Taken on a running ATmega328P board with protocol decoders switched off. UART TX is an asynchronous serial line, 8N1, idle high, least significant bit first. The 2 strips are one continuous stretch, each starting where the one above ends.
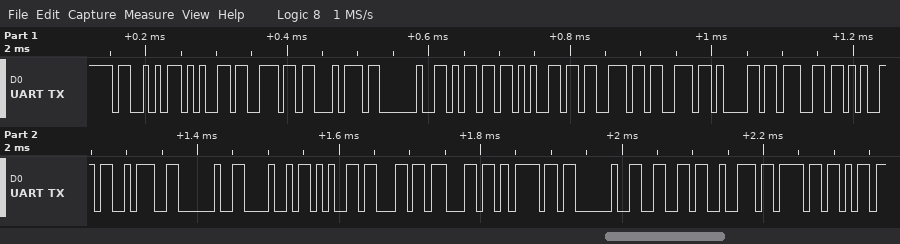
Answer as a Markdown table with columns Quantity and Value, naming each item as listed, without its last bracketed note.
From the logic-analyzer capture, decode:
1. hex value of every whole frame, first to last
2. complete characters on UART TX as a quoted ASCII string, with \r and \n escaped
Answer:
| Quantity | Value |
|---|---|
| hex value of every whole frame, first to last | 0x53 0x65 0x6E 0x74 0x20 0x6D 0x65 0x73 0x73 0x61 0x67 0x65 0x3A 0x20 0x48 0x65 0x6C 0x6C 0x6F 0x20 0x66 0x72 0x6F |
| complete characters on UART TX as a quoted ASCII string, with \r and \n escaped | "Sent message: Hello fro" |
